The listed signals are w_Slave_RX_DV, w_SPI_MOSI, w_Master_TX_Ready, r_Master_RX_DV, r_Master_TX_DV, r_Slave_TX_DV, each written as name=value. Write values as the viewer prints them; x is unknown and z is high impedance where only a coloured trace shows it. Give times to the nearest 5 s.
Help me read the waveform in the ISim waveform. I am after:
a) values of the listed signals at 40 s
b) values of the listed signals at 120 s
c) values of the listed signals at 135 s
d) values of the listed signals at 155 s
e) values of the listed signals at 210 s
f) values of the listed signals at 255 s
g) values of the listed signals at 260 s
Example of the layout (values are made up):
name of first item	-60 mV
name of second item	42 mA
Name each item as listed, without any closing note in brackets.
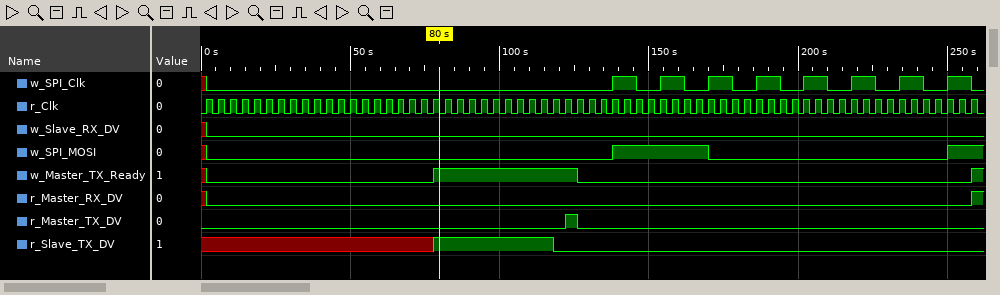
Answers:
values of the listed signals at 40 s	w_Slave_RX_DV=0, w_SPI_MOSI=0, w_Master_TX_Ready=0, r_Master_RX_DV=0, r_Master_TX_DV=0, r_Slave_TX_DV=x
values of the listed signals at 120 s	w_Slave_RX_DV=0, w_SPI_MOSI=0, w_Master_TX_Ready=1, r_Master_RX_DV=0, r_Master_TX_DV=0, r_Slave_TX_DV=0
values of the listed signals at 135 s	w_Slave_RX_DV=0, w_SPI_MOSI=0, w_Master_TX_Ready=0, r_Master_RX_DV=0, r_Master_TX_DV=0, r_Slave_TX_DV=0
values of the listed signals at 155 s	w_Slave_RX_DV=0, w_SPI_MOSI=1, w_Master_TX_Ready=0, r_Master_RX_DV=0, r_Master_TX_DV=0, r_Slave_TX_DV=0
values of the listed signals at 210 s	w_Slave_RX_DV=0, w_SPI_MOSI=0, w_Master_TX_Ready=0, r_Master_RX_DV=0, r_Master_TX_DV=0, r_Slave_TX_DV=0
values of the listed signals at 255 s	w_Slave_RX_DV=0, w_SPI_MOSI=1, w_Master_TX_Ready=0, r_Master_RX_DV=0, r_Master_TX_DV=0, r_Slave_TX_DV=0
values of the listed signals at 260 s	w_Slave_RX_DV=0, w_SPI_MOSI=1, w_Master_TX_Ready=1, r_Master_RX_DV=1, r_Master_TX_DV=0, r_Slave_TX_DV=0
